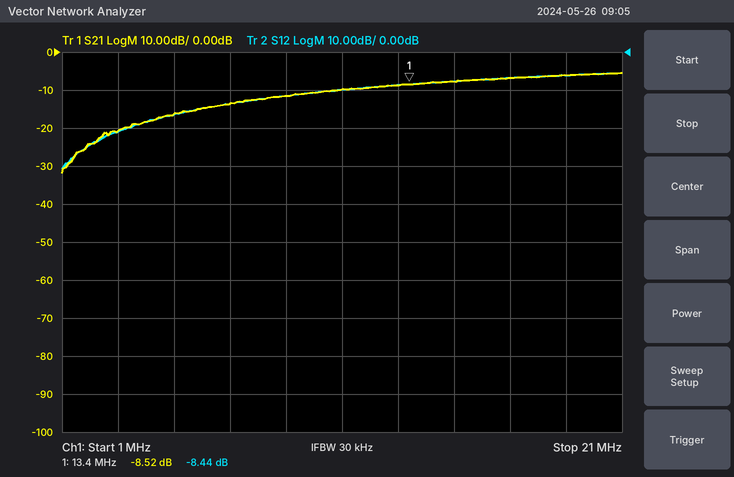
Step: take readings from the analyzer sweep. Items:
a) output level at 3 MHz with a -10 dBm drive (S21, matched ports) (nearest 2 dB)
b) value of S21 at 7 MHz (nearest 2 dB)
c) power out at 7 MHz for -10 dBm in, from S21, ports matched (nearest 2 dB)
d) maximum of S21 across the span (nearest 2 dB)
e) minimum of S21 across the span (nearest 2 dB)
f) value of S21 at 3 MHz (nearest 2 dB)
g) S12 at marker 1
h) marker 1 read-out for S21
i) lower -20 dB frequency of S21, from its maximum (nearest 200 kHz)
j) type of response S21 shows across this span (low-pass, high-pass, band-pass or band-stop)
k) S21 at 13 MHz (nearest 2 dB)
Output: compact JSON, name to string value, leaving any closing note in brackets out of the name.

{"output level at 3 MHz with a -10 dBm drive (S21, matched ports)": "-30 dBm", "value of S21 at 7 MHz": "-14 dB", "power out at 7 MHz for -10 dBm in, from S21, ports matched": "-24 dBm", "maximum of S21 across the span": "-6 dB", "minimum of S21 across the span": "-32 dB", "value of S21 at 3 MHz": "-20 dB", "S12 at marker 1": "-8.44 dB", "marker 1 read-out for S21": "-8.52 dB", "lower -20 dB frequency of S21, from its maximum": "1.8 MHz", "type of response S21 shows across this span": "high-pass", "S21 at 13 MHz": "-8 dB"}
